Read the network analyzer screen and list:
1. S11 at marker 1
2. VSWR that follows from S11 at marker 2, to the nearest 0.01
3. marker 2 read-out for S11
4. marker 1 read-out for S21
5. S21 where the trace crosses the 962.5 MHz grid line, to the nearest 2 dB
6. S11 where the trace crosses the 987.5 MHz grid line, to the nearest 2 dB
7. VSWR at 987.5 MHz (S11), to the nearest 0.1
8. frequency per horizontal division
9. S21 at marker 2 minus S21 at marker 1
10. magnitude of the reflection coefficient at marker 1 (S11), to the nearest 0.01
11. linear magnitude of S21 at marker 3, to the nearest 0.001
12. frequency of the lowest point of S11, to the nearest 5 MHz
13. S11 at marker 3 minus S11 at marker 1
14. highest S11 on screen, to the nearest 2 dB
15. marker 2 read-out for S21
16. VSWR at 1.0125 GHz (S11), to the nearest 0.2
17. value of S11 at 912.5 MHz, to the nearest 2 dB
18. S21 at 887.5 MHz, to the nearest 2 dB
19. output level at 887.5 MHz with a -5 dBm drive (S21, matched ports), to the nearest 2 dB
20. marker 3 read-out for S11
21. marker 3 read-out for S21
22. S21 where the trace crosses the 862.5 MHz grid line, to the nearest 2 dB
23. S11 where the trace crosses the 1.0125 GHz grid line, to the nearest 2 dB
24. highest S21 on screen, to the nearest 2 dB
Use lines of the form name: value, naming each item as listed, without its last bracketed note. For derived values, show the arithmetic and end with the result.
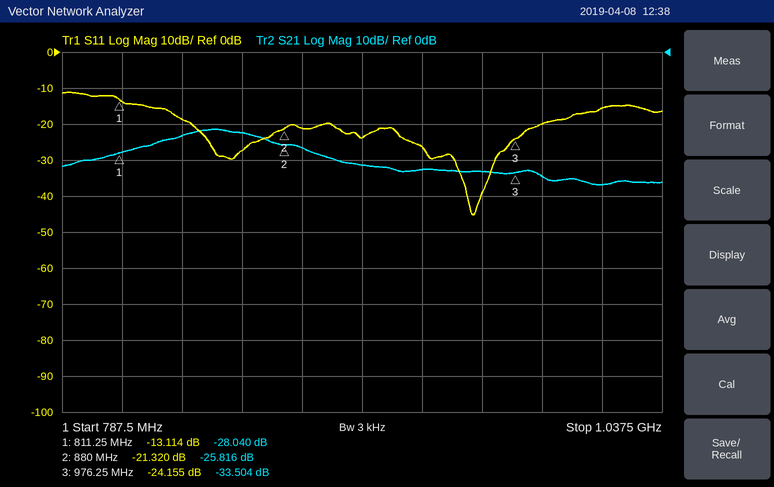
S11 at marker 1: -13.114 dB
VSWR that follows from S11 at marker 2, to the nearest 0.01: (1 + 0.0859)/(1 − 0.0859) ≈ 1.19
marker 2 read-out for S11: -21.320 dB
marker 1 read-out for S21: -28.040 dB
S21 where the trace crosses the 962.5 MHz grid line, to the nearest 2 dB: -34 dB
S11 where the trace crosses the 987.5 MHz grid line, to the nearest 2 dB: -20 dB
VSWR at 987.5 MHz (S11), to the nearest 0.1: |Γ| = 10^(-20/20) = 0.1000; VSWR = (1 + 0.1000)/(1 − 0.1000) ≈ 1.2
frequency per horizontal division: 25 MHz
S21 at marker 2 minus S21 at marker 1: -25.816 − (-28.04) = 2.224 dB
magnitude of the reflection coefficient at marker 1 (S11), to the nearest 0.01: 10^(-13.114/20) ≈ 0.22
linear magnitude of S21 at marker 3, to the nearest 0.001: 10^(-33.504/20) ≈ 0.021
frequency of the lowest point of S11, to the nearest 5 MHz: 960 MHz
S11 at marker 3 minus S11 at marker 1: -24.155 − (-13.114) = -11.041 dB
highest S11 on screen, to the nearest 2 dB: -12 dB
marker 2 read-out for S21: -25.816 dB
VSWR at 1.0125 GHz (S11), to the nearest 0.2: |Γ| = 10^(-16/20) = 0.1585; VSWR = (1 + 0.1585)/(1 − 0.1585) ≈ 1.4
value of S11 at 912.5 MHz, to the nearest 2 dB: -24 dB
S21 at 887.5 MHz, to the nearest 2 dB: -26 dB
output level at 887.5 MHz with a -5 dBm drive (S21, matched ports), to the nearest 2 dB: -5 dBm + (-26 dB) = -32 dBm
marker 3 read-out for S11: -24.155 dB
marker 3 read-out for S21: -33.504 dB
S21 where the trace crosses the 862.5 MHz grid line, to the nearest 2 dB: -22 dB
S11 where the trace crosses the 1.0125 GHz grid line, to the nearest 2 dB: -16 dB
highest S21 on screen, to the nearest 2 dB: -22 dB
